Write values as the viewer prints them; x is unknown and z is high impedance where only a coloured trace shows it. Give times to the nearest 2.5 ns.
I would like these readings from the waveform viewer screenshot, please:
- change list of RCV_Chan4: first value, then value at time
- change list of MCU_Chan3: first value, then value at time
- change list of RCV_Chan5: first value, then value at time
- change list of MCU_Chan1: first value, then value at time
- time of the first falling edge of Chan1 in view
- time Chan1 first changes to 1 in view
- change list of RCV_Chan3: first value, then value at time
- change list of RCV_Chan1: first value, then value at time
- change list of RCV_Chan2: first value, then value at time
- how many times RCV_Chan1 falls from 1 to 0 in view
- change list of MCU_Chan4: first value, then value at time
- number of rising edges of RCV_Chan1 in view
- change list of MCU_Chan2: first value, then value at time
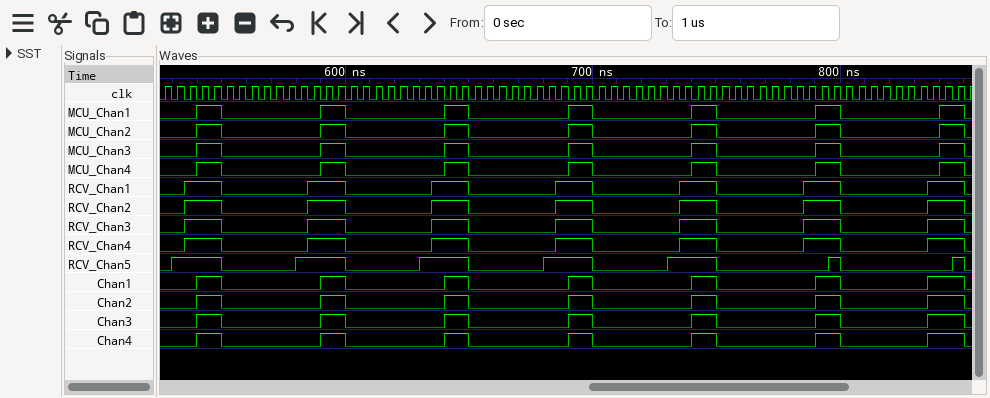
0, 1 at 535 ns, 0 at 550 ns, 1 at 585 ns, 0 at 600 ns, 1 at 635 ns, 0 at 650 ns, 1 at 685 ns, 0 at 700 ns, 1 at 735 ns, 0 at 750 ns, 1 at 785 ns, 0 at 800 ns, 1 at 835 ns, 0 at 850 ns
0, 1 at 540 ns, 0 at 550 ns, 1 at 590 ns, 0 at 600 ns, 1 at 640 ns, 0 at 650 ns, 1 at 690 ns, 0 at 700 ns, 1 at 740 ns, 0 at 750 ns, 1 at 790 ns, 0 at 800 ns, 1 at 840 ns, 0 at 850 ns
0, 1 at 530 ns, 0 at 550 ns, 1 at 580 ns, 0 at 600 ns, 1 at 630 ns, 0 at 650 ns, 1 at 680 ns, 0 at 700 ns, 1 at 730 ns, 0 at 750 ns, 1 at 795 ns, 0 at 800 ns, 1 at 845 ns, 0 at 850 ns
0, 1 at 540 ns, 0 at 550 ns, 1 at 590 ns, 0 at 600 ns, 1 at 640 ns, 0 at 650 ns, 1 at 690 ns, 0 at 700 ns, 1 at 740 ns, 0 at 750 ns, 1 at 790 ns, 0 at 800 ns, 1 at 840 ns, 0 at 850 ns
550 ns
540 ns
0, 1 at 535 ns, 0 at 550 ns, 1 at 585 ns, 0 at 600 ns, 1 at 635 ns, 0 at 650 ns, 1 at 685 ns, 0 at 700 ns, 1 at 735 ns, 0 at 750 ns, 1 at 785 ns, 0 at 800 ns, 1 at 835 ns, 0 at 850 ns
0, 1 at 535 ns, 0 at 550 ns, 1 at 585 ns, 0 at 600 ns, 1 at 635 ns, 0 at 650 ns, 1 at 685 ns, 0 at 700 ns, 1 at 735 ns, 0 at 750 ns, 1 at 785 ns, 0 at 800 ns, 1 at 835 ns, 0 at 850 ns
0, 1 at 535 ns, 0 at 550 ns, 1 at 585 ns, 0 at 600 ns, 1 at 635 ns, 0 at 650 ns, 1 at 685 ns, 0 at 700 ns, 1 at 735 ns, 0 at 750 ns, 1 at 785 ns, 0 at 800 ns, 1 at 835 ns, 0 at 850 ns
7
0, 1 at 540 ns, 0 at 550 ns, 1 at 590 ns, 0 at 600 ns, 1 at 640 ns, 0 at 650 ns, 1 at 690 ns, 0 at 700 ns, 1 at 740 ns, 0 at 750 ns, 1 at 790 ns, 0 at 800 ns, 1 at 840 ns, 0 at 850 ns
7
0, 1 at 540 ns, 0 at 550 ns, 1 at 590 ns, 0 at 600 ns, 1 at 640 ns, 0 at 650 ns, 1 at 690 ns, 0 at 700 ns, 1 at 740 ns, 0 at 750 ns, 1 at 790 ns, 0 at 800 ns, 1 at 840 ns, 0 at 850 ns
